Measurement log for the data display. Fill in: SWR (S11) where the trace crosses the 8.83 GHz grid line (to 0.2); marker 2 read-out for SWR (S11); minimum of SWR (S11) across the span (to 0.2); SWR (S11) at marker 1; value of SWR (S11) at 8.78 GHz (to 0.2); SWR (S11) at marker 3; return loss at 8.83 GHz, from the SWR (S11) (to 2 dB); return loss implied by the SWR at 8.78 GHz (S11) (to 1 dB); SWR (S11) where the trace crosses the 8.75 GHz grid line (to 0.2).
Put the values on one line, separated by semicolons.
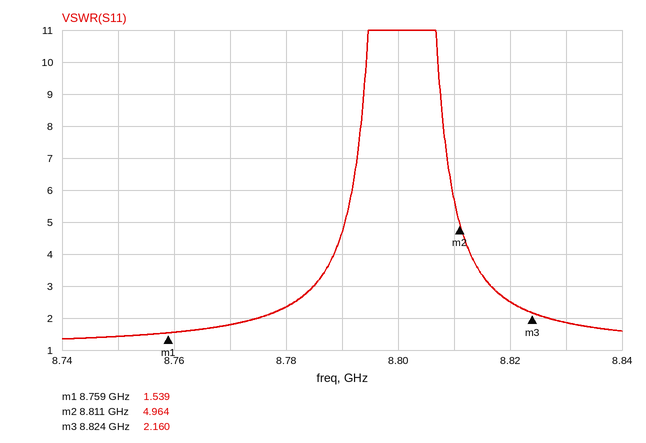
1.8; 4.964; 1.4; 1.539; 2.4; 2.160; 10 dB; 8 dB; 1.4
